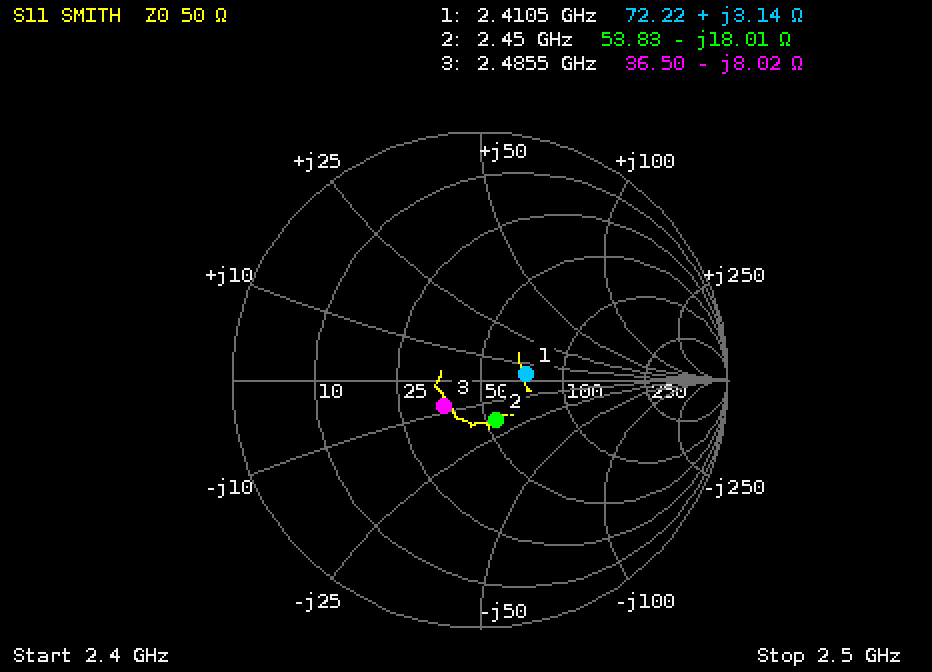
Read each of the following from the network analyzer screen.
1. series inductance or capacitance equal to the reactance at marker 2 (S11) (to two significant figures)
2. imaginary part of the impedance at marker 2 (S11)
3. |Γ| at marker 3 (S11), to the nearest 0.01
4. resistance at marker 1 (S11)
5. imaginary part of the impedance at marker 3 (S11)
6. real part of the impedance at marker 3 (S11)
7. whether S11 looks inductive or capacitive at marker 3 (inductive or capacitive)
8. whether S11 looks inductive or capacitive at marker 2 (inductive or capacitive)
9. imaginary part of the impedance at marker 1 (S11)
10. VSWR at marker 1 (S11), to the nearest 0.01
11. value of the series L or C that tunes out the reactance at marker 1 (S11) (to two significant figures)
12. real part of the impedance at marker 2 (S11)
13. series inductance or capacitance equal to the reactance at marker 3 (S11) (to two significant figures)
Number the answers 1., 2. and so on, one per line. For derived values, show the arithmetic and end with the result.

1. C = 1/(2π × 2.45 GHz × 18.01 Ω) ≈ 3.6 pF
2. -18.01 Ω
3. 0.18
4. 72.22 Ω
5. -8.02 Ω
6. 36.50 Ω
7. capacitive
8. capacitive
9. +3.14 Ω
10. 1.45
11. C = 1/(2π × 2.4105 GHz × 3.14 Ω) ≈ 21 pF
12. 53.83 Ω
13. C = 1/(2π × 2.4855 GHz × 8.02 Ω) ≈ 8.0 pF
